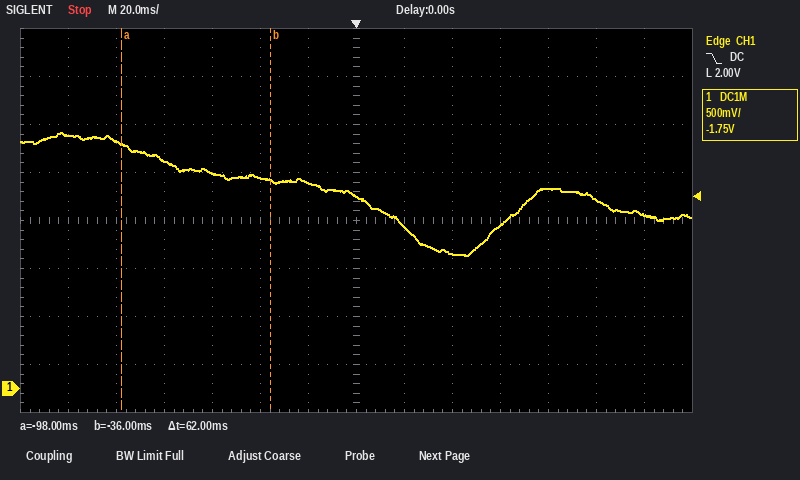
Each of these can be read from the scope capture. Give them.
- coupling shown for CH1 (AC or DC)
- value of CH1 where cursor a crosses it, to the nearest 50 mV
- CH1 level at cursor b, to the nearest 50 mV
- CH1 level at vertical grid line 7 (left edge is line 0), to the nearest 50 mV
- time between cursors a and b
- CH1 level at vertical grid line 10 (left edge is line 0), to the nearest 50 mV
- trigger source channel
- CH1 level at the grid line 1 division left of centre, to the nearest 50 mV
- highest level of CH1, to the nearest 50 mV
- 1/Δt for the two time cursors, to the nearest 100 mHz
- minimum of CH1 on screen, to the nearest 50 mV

DC
2.55 V
2.15 V
2.00 V
62 ms
1.70 V
CH1
2.15 V
2.65 V
16.1 Hz
1.40 V
